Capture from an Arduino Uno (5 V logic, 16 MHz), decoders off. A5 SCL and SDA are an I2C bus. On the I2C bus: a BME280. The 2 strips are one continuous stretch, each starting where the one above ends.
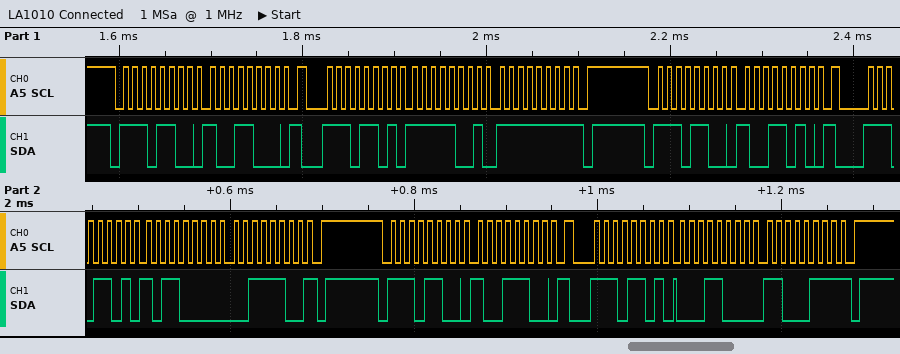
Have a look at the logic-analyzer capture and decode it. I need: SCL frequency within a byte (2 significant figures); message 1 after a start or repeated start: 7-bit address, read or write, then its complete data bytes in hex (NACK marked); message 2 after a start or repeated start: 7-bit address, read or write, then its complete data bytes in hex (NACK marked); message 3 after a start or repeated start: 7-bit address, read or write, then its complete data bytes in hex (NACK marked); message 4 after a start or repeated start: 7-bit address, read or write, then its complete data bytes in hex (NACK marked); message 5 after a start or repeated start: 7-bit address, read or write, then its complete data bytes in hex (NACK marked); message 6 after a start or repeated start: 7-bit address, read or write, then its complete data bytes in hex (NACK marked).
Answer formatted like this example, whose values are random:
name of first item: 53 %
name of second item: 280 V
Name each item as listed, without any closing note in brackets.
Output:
SCL frequency within a byte: 100 kHz
message 1 after a start or repeated start: 7-bit address, read or write, then its complete data bytes in hex: 0x76 write: 98
message 2 after a start or repeated start: 7-bit address, read or write, then its complete data bytes in hex: 0x76 read: F9 FF NACK
message 3 after a start or repeated start: 7-bit address, read or write, then its complete data bytes in hex: 0x76 write: 9A
message 4 after a start or repeated start: 7-bit address, read or write, then its complete data bytes in hex: 0x76 read: B0 3C NACK
message 5 after a start or repeated start: 7-bit address, read or write, then its complete data bytes in hex: 0x76 write: 9C
message 6 after a start or repeated start: 7-bit address, read or write, then its complete data bytes in hex: 0x76 read: 18 C7 NACK
